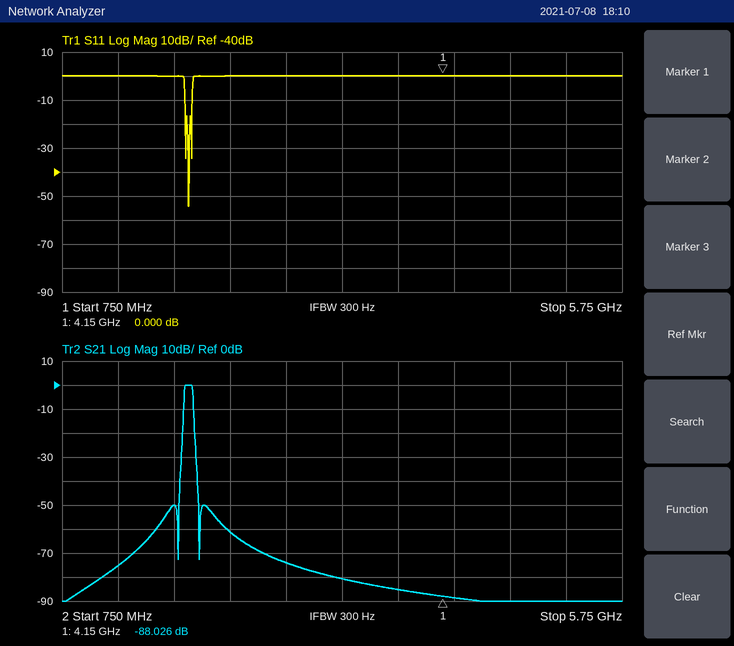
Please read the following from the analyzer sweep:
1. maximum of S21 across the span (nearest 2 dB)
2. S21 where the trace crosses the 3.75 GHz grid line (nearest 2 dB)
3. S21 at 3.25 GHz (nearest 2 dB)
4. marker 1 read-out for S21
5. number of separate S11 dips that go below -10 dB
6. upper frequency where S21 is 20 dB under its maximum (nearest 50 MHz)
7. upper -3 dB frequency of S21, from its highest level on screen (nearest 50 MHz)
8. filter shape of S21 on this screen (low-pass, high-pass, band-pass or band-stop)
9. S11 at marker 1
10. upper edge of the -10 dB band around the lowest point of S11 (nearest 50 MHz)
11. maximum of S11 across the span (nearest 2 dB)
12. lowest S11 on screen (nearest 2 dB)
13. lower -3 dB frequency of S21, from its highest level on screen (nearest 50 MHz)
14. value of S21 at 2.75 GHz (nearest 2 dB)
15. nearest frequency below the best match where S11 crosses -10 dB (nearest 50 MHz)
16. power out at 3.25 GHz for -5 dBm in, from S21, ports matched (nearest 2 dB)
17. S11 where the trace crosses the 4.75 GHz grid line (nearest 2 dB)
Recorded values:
0 dB
-86 dB
-80 dB
-88.026 dB
3
1.95 GHz
1.90 GHz
band-pass
0.000 dB
1.90 GHz
0 dB
-54 dB
1.85 GHz
-74 dB
1.85 GHz
-86 dBm
0 dB
